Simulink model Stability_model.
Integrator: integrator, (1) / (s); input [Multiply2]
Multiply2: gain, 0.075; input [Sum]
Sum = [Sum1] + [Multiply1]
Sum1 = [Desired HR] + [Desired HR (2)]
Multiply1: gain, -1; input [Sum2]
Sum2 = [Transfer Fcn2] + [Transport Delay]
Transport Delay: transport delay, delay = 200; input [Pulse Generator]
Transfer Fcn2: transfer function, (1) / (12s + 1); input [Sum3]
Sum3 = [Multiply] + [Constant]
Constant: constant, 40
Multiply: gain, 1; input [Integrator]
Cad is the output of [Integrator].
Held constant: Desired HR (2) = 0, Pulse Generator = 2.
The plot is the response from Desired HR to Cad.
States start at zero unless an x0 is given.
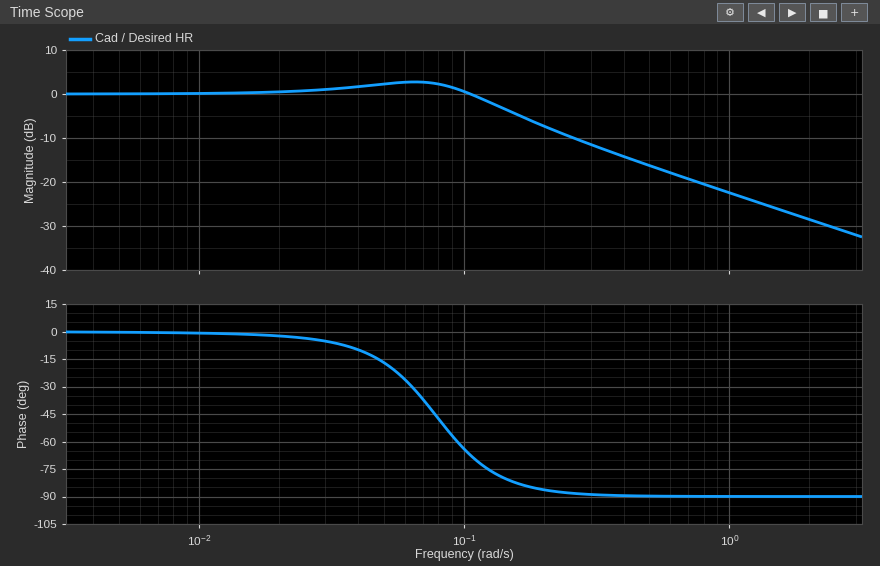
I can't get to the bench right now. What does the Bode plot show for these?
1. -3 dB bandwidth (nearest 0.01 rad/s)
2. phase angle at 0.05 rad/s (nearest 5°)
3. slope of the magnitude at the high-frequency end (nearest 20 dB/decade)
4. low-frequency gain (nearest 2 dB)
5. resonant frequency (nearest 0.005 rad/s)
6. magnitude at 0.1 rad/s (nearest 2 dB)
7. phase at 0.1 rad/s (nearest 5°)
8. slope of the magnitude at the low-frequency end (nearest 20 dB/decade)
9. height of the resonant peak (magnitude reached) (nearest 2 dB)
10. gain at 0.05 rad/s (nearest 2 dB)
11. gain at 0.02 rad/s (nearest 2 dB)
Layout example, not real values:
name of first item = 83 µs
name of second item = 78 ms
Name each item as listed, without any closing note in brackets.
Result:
-3 dB bandwidth = 0.14 rad/s
phase angle at 0.05 rad/s = -15°
slope of the magnitude at the high-frequency end = -20 dB/decade
low-frequency gain = 0 dB
resonant frequency = 0.065 rad/s
magnitude at 0.1 rad/s = 0 dB
phase at 0.1 rad/s = -65°
slope of the magnitude at the low-frequency end = 0 dB/decade
height of the resonant peak (magnitude reached) = 2 dB
gain at 0.05 rad/s = 2 dB
gain at 0.02 rad/s = 0 dB
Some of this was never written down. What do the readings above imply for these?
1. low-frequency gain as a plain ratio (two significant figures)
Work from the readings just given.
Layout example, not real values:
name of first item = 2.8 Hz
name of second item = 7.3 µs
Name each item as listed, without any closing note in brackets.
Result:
low-frequency gain as a plain ratio = 1.0
